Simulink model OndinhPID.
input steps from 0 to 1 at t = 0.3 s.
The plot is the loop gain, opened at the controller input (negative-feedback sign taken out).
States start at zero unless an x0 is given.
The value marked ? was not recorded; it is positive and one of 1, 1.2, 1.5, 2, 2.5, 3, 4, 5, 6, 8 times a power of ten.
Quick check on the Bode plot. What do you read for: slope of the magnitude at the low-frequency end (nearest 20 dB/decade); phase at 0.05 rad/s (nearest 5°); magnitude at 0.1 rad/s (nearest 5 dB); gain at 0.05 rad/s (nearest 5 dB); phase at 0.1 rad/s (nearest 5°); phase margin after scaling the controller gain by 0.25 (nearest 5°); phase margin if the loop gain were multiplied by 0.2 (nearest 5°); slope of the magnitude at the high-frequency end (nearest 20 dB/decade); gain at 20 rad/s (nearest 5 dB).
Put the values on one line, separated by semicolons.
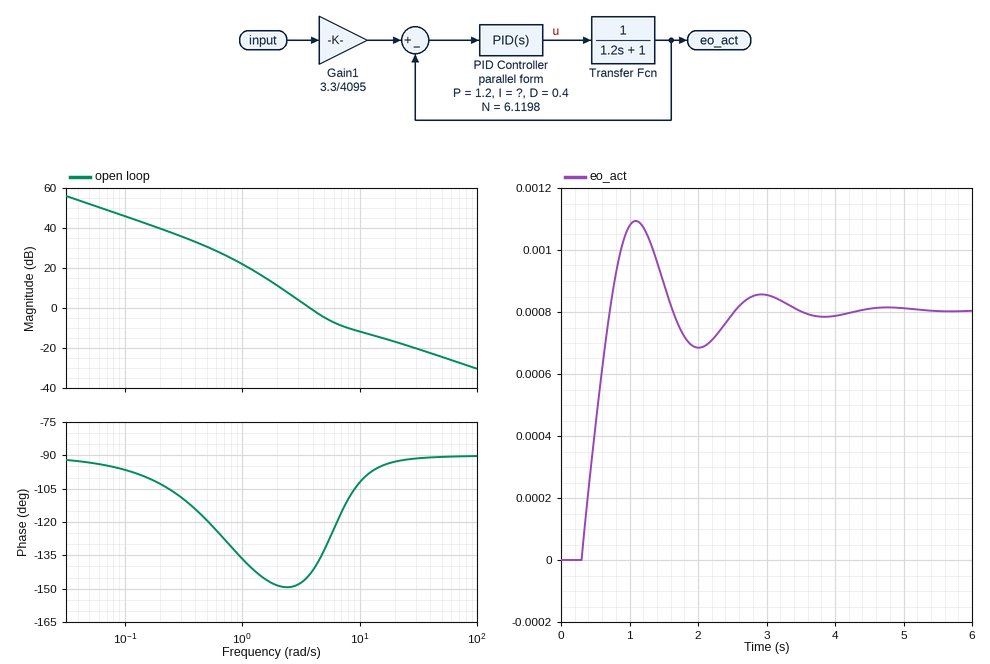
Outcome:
-20 dB/decade; -95°; 45 dB; 50 dB; -95°; 30°; 35°; -20 dB/decade; -15 dB
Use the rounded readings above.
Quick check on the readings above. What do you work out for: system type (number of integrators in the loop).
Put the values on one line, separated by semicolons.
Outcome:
1
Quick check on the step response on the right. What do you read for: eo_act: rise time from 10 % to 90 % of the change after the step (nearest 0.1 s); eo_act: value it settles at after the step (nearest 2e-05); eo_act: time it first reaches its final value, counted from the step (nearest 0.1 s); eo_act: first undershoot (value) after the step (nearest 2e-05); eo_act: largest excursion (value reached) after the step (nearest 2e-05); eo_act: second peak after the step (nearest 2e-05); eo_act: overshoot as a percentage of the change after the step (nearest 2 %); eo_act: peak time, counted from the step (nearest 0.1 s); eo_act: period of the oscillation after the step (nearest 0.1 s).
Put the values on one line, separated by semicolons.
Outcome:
0.3 s; 0.00080; 0.4 s; 0.00068; 0.00110; 0.00086; 36 %; 0.8 s; 1.8 s
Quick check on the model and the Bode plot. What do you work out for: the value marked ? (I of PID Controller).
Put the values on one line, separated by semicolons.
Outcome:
20
